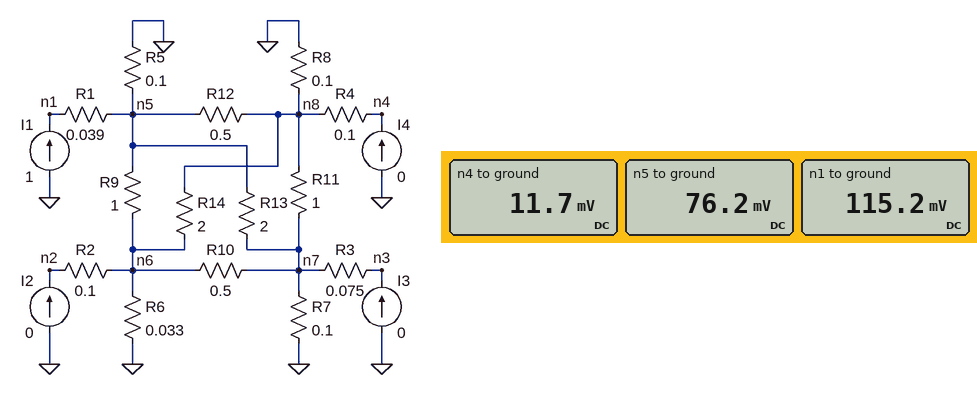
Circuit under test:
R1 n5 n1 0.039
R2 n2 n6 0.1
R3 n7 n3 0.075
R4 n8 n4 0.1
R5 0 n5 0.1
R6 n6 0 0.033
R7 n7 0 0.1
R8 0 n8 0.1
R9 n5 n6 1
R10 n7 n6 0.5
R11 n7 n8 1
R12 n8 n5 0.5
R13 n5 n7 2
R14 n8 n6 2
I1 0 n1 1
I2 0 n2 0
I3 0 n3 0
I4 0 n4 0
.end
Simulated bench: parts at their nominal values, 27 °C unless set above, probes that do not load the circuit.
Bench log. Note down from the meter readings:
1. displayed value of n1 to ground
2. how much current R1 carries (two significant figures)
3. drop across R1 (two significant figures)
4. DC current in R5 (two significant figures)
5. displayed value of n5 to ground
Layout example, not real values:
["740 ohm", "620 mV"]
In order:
["115.2 mV", "1.0 A", "39 mV", "760 mA", "76.2 mV"]
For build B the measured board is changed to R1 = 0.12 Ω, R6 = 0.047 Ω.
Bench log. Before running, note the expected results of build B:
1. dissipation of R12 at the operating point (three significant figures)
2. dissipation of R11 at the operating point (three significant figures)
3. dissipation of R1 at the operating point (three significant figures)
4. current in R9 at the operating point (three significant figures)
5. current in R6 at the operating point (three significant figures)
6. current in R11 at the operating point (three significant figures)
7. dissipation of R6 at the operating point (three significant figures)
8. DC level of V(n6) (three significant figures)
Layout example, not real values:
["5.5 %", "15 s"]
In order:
["8.32 mW", "56.4 µW", "120 mW", "72.6 mA", "77.8 mA", "7.51 mA", "284 µW", "3.66 mV"]
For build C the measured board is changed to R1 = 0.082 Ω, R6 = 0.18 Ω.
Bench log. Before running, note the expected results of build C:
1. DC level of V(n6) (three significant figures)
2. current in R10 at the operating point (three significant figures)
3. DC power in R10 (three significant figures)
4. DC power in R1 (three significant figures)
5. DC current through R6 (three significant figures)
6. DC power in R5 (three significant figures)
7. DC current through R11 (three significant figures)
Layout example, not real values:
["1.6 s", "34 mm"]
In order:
["10.3 mV", "10.1 mA", "50.9 µW", "82.0 mW", "57.3 mA", "59.0 mW", "6.88 mA"]
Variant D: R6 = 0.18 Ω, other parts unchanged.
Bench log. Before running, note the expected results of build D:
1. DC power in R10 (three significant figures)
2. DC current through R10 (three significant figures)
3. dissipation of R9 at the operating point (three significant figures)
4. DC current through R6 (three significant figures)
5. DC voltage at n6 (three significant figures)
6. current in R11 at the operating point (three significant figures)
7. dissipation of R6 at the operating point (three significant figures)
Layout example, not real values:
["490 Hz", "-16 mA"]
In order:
["50.9 µW", "10.1 mA", "4.42 mW", "57.3 mA", "10.3 mV", "6.88 mA", "592 µW"]
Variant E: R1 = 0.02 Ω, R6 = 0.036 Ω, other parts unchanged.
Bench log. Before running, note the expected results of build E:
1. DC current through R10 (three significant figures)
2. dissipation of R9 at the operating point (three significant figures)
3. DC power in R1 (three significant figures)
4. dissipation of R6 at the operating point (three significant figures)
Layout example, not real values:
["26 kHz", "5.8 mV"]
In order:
["2.46 mA", "5.37 mW", "20.0 mW", "231 µW"]
